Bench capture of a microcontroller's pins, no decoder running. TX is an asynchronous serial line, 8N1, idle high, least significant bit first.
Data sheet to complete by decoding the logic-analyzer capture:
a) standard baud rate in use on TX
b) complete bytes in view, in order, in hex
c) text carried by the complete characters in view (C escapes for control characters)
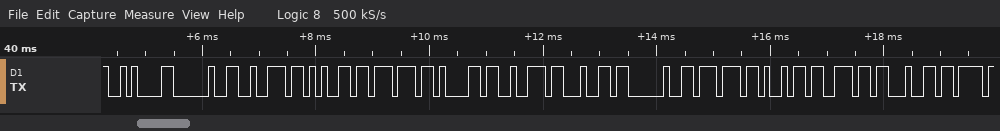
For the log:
9600 baud
0A 20 72 65 77 61 72 64 20 77 69 6E 64
"\n reward wind"
